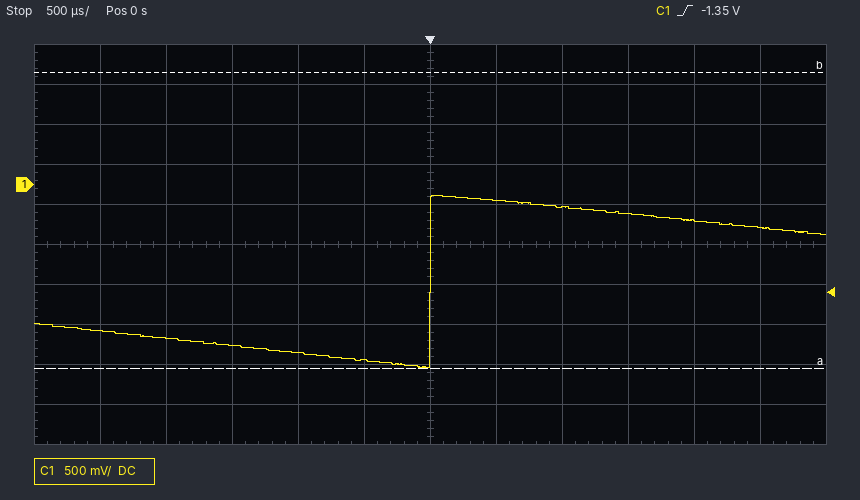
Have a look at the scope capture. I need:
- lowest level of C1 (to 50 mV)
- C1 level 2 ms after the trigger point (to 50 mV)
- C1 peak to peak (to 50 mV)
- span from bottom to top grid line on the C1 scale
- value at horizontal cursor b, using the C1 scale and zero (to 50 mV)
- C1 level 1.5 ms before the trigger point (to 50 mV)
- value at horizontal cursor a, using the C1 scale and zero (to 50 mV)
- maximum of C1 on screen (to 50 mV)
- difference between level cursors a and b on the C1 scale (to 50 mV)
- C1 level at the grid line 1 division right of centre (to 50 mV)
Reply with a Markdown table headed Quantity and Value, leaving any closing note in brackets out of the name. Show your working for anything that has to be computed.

| Quantity | Value |
|---|---|
| lowest level of C1 | -2.30 V |
| C1 level 2 ms after the trigger point | -450 mV |
| C1 peak to peak | -150 mV − (-2.30 V) = 2.15 V |
| span from bottom to top grid line on the C1 scale | 5 V |
| value at horizontal cursor b, using the C1 scale and zero | 1.40 V |
| C1 level 1.5 ms before the trigger point | -2.00 V |
| value at horizontal cursor a, using the C1 scale and zero | -2.30 V |
| maximum of C1 on screen | -150 mV |
| difference between level cursors a and b on the C1 scale | 3.70 V |
| C1 level at the grid line 1 division right of centre | -200 mV |
